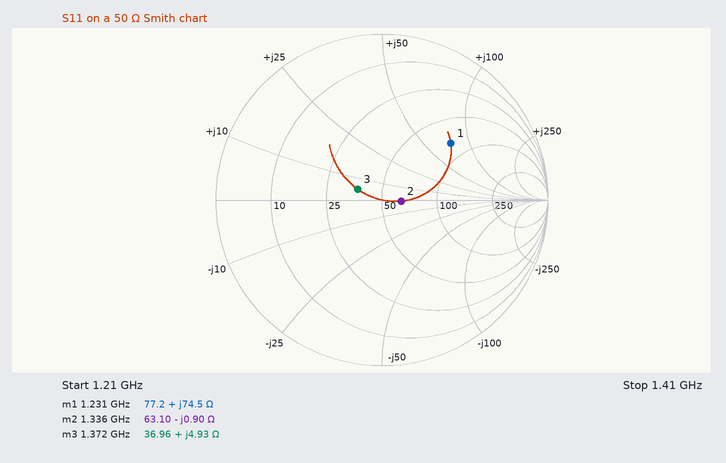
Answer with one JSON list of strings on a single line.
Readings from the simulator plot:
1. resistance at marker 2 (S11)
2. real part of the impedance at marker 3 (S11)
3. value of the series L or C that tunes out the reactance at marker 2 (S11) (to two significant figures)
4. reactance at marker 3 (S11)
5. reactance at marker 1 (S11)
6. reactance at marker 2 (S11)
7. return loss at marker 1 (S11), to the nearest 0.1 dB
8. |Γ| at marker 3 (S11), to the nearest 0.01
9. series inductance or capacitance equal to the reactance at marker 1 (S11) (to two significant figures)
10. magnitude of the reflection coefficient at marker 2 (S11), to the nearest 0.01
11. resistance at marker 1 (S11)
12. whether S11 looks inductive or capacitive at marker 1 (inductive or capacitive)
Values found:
["63.10 Ω", "36.96 Ω", "110 pH", "+4.93 Ω", "+74.5 Ω", "-0.90 Ω", "5.4 dB", "0.16", "9.6 nH", "0.12", "77.2 Ω", "inductive"]
